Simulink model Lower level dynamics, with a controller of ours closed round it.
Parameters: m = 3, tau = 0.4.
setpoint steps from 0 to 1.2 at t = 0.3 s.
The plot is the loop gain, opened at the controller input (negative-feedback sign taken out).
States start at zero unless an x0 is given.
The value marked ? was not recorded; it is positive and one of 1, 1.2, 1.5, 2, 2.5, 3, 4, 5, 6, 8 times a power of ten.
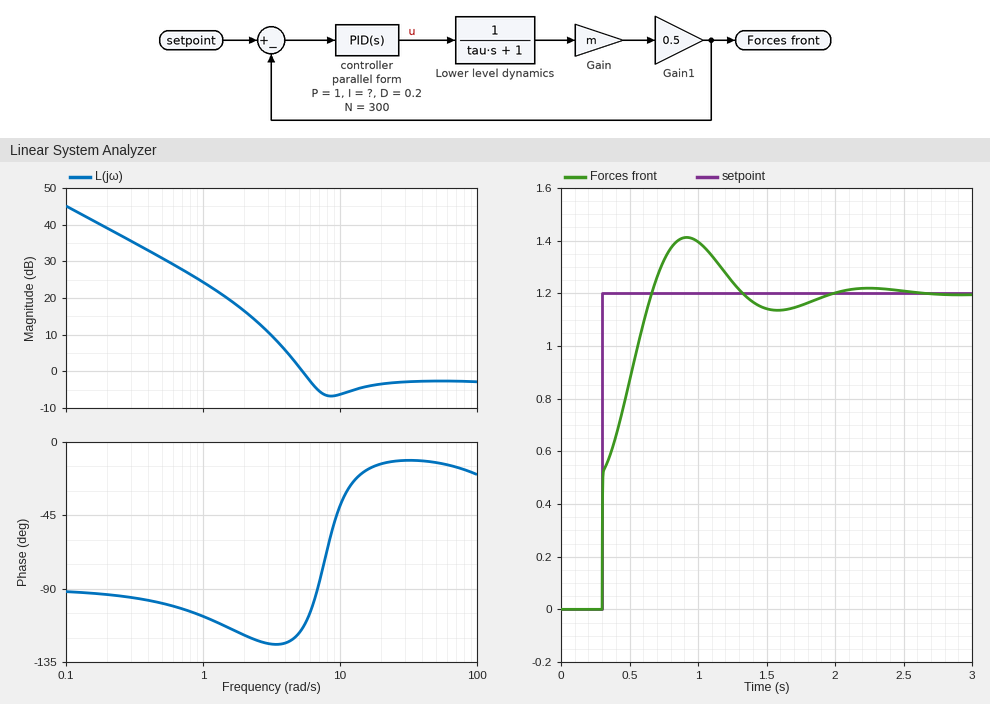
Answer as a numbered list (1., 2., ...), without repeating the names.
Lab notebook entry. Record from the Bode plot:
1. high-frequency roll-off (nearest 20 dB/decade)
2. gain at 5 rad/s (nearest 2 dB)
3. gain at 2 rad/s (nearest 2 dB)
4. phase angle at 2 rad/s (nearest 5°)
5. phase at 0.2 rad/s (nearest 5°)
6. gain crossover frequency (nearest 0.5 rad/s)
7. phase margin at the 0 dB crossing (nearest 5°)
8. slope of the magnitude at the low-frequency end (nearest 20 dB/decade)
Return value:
1. 0 dB/decade
2. 2 dB
3. 16 dB
4. -120°
5. -95°
6. 5.5 rad/s
7. 65°
8. -20 dB/decade
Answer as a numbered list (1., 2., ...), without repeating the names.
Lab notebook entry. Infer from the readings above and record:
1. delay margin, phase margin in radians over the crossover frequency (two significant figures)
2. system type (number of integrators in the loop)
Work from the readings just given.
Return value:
1. 0.21 s
2. 1
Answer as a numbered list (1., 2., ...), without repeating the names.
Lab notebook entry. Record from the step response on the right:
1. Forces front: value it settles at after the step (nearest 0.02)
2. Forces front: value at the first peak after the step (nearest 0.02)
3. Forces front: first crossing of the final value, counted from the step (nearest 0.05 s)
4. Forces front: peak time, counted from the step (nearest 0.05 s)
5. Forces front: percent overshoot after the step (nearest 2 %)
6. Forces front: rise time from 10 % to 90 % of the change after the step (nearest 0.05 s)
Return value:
1. 1.20
2. 1.42
3. 0.35 s
4. 0.60 s
5. 18 %
6. 0.30 s
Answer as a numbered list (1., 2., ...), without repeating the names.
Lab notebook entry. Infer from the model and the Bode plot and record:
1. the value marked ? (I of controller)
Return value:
1. 12
